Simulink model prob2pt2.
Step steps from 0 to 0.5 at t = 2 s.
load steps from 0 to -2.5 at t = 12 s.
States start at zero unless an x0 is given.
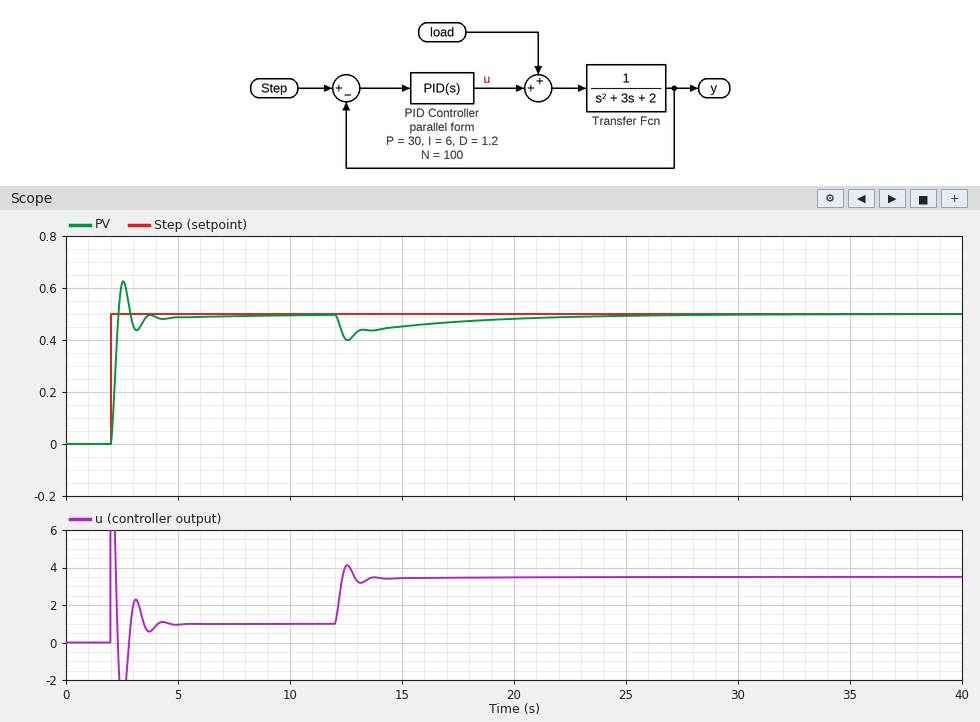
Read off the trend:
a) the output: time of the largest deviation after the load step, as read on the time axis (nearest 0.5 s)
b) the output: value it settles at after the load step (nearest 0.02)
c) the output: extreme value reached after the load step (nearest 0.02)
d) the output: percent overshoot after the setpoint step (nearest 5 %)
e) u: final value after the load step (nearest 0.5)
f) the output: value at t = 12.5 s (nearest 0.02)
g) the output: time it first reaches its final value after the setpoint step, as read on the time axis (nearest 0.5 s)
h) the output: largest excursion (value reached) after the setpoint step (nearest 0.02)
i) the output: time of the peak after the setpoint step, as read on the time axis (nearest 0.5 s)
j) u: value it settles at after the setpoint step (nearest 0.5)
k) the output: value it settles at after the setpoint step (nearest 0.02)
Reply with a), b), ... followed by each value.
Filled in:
a) 12.5 s
b) 0.50
c) 0.40
d) 25 %
e) 3.5
f) 0.40
g) 2.5 s
h) 0.62
i) 2.5 s
j) 1.0
k) 0.50
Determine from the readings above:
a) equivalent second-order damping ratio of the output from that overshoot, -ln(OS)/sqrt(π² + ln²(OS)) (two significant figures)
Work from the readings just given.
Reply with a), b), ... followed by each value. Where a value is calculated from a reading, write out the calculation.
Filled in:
a) ln(0.25) = -1.386; 1.386 / sqrt(9.870 + 1.922) = 0.40
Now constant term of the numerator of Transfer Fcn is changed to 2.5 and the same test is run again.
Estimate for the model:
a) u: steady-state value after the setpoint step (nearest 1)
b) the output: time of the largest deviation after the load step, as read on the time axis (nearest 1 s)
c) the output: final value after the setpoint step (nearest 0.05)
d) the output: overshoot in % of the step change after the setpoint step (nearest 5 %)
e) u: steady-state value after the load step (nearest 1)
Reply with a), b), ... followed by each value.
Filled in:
a) 0
b) 12 s
c) 0.50
d) 35 %
e) 3
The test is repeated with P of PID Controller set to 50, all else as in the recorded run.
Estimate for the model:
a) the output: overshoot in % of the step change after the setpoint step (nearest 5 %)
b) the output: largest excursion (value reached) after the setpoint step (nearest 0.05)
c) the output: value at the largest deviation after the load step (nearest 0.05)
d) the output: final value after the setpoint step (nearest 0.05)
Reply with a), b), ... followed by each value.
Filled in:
a) 35 %
b) 0.70
c) 0.45
d) 0.50
